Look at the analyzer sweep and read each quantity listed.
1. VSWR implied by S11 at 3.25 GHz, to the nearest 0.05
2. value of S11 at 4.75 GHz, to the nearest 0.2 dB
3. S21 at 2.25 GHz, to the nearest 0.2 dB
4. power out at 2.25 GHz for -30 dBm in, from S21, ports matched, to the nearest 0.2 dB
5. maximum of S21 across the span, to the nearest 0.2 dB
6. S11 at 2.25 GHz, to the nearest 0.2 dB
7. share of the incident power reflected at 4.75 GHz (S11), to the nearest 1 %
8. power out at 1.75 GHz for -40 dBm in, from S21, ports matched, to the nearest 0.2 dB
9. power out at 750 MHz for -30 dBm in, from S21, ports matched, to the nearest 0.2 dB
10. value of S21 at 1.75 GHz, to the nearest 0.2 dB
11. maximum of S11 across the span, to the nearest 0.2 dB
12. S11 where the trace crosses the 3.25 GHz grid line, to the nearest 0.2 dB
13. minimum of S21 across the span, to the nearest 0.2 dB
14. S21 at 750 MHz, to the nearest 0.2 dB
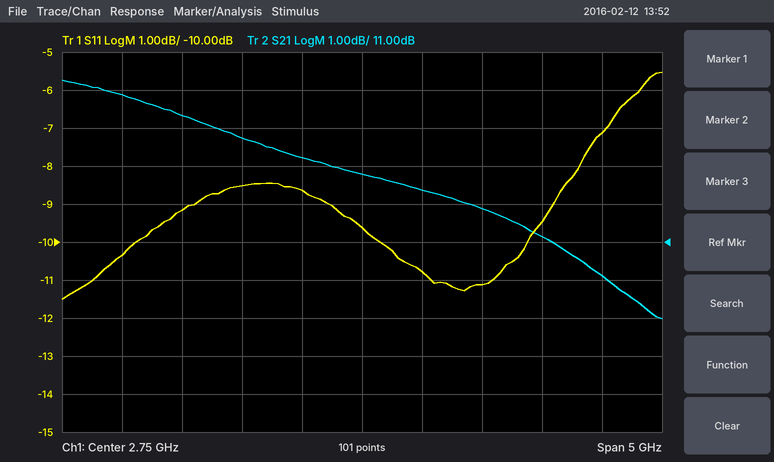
1.80
-7.2 dB
13.2 dB
-16.8 dBm
15.2 dB
-8.6 dB
19 %
-26.2 dBm
-15.2 dBm
13.8 dB
-5.6 dB
-10.8 dB
9.0 dB
14.8 dB
